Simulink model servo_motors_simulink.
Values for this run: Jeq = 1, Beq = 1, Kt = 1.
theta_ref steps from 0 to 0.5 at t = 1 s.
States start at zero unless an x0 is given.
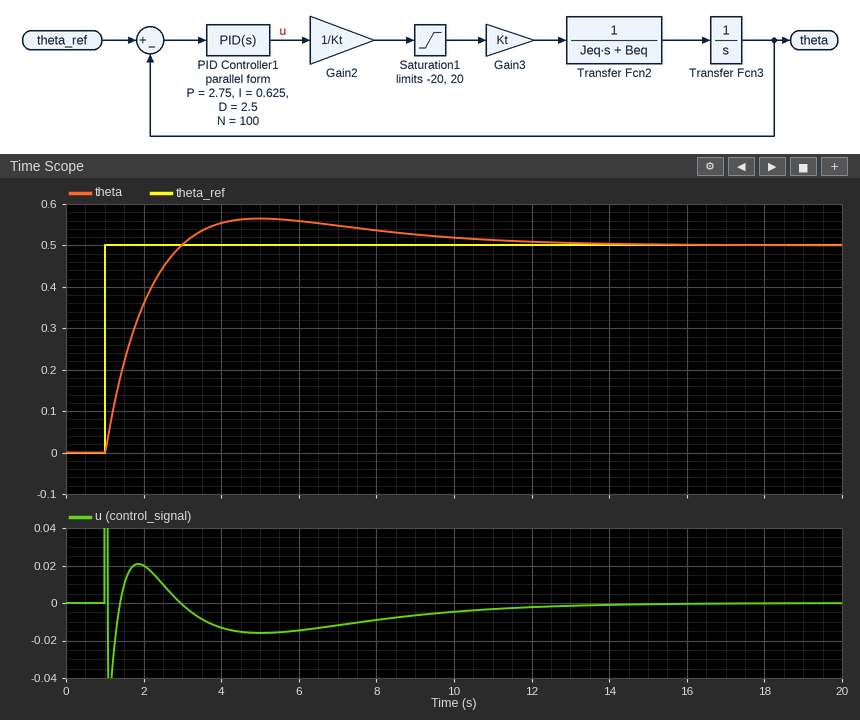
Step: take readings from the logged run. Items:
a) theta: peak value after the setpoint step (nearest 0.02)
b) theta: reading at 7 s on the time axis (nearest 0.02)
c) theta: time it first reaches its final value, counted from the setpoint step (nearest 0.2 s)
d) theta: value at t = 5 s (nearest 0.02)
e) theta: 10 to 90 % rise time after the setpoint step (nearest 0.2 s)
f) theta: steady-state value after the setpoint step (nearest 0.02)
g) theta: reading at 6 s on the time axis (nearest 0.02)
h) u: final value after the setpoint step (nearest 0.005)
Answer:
0.56
0.54
2.0 s
0.56
1.4 s
0.50
0.56
0.000
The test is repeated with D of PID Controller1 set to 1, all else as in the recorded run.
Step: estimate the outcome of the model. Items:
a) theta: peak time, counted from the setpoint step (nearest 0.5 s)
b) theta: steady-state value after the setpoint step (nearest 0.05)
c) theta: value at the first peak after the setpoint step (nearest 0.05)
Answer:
2.0 s
0.50
0.60
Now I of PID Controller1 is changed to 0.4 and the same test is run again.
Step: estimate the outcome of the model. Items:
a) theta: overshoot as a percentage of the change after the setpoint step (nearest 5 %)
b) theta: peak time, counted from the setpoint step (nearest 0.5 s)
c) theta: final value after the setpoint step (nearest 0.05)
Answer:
10 %
4.5 s
0.50
